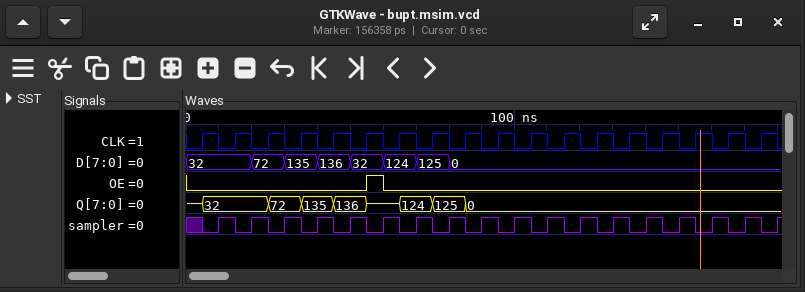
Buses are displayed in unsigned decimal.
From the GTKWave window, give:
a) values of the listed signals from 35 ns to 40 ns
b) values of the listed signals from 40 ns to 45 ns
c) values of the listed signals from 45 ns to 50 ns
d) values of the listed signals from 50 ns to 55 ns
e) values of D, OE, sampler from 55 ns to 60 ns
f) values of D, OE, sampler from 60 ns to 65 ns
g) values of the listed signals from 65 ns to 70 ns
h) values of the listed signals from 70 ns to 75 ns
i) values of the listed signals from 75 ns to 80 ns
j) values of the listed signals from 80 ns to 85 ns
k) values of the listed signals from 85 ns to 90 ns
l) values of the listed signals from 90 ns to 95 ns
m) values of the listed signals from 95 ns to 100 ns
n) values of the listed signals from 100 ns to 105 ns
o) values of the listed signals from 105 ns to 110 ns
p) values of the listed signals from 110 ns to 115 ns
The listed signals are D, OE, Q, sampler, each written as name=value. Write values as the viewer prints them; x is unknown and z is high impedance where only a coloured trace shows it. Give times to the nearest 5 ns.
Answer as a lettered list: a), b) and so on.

a) D=135, OE=0, Q=135, sampler=0
b) D=136, OE=0, Q=135, sampler=1
c) D=136, OE=0, Q=136, sampler=0
d) D=32, OE=0, Q=136, sampler=1
e) D=32, OE=1, sampler=0
f) D=124, OE=0, sampler=1
g) D=124, OE=0, Q=124, sampler=0
h) D=125, OE=0, Q=124, sampler=1
i) D=125, OE=0, Q=125, sampler=0
j) D=0, OE=0, Q=125, sampler=1
k) D=0, OE=0, Q=0, sampler=0
l) D=0, OE=0, Q=0, sampler=1
m) D=0, OE=0, Q=0, sampler=0
n) D=0, OE=0, Q=0, sampler=1
o) D=0, OE=0, Q=0, sampler=0
p) D=0, OE=0, Q=0, sampler=1
